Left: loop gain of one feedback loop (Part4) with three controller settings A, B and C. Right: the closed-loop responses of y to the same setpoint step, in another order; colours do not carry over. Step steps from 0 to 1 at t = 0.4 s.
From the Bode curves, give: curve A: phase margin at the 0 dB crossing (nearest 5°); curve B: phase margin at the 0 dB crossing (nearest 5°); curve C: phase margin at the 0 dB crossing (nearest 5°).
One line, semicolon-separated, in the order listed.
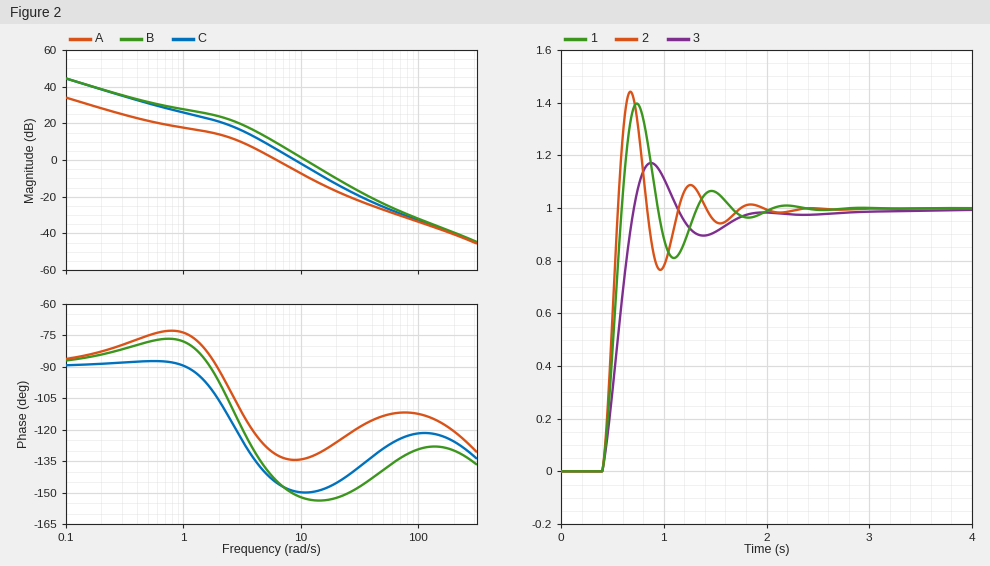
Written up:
50°; 25°; 30°
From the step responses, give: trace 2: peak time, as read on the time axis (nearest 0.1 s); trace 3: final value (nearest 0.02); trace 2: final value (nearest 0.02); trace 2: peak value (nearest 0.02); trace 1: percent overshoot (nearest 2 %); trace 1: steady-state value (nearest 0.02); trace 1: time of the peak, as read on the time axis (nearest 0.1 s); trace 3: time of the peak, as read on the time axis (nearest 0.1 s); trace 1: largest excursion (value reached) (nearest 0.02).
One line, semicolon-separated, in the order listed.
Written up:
0.7 s; 1.00; 1.00; 1.44; 40 %; 1.00; 0.7 s; 0.9 s; 1.40
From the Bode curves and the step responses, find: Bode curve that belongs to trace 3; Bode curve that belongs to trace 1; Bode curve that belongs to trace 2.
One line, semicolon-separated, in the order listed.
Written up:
A; C; B
